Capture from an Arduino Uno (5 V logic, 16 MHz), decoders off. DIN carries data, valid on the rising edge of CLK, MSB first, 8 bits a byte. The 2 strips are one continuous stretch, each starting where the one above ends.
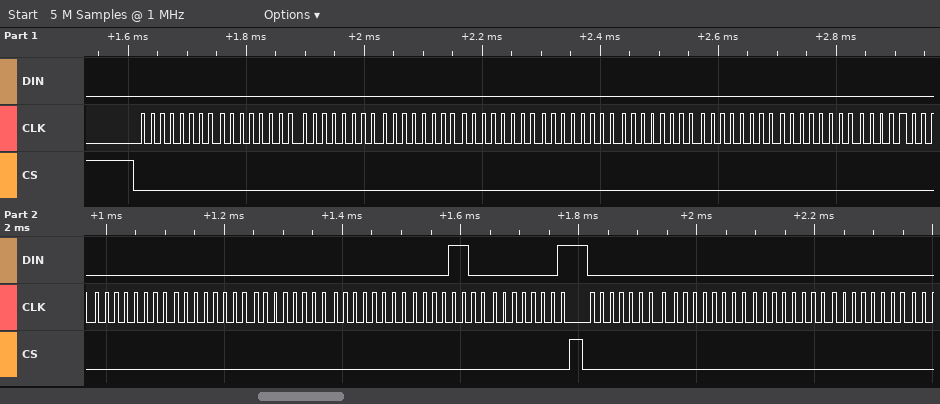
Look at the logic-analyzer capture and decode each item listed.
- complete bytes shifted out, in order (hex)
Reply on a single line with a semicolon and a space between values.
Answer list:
00 00 00 00 00 00 00 00 00 00 00 00 00 00 0C 01 00 00 00 00
